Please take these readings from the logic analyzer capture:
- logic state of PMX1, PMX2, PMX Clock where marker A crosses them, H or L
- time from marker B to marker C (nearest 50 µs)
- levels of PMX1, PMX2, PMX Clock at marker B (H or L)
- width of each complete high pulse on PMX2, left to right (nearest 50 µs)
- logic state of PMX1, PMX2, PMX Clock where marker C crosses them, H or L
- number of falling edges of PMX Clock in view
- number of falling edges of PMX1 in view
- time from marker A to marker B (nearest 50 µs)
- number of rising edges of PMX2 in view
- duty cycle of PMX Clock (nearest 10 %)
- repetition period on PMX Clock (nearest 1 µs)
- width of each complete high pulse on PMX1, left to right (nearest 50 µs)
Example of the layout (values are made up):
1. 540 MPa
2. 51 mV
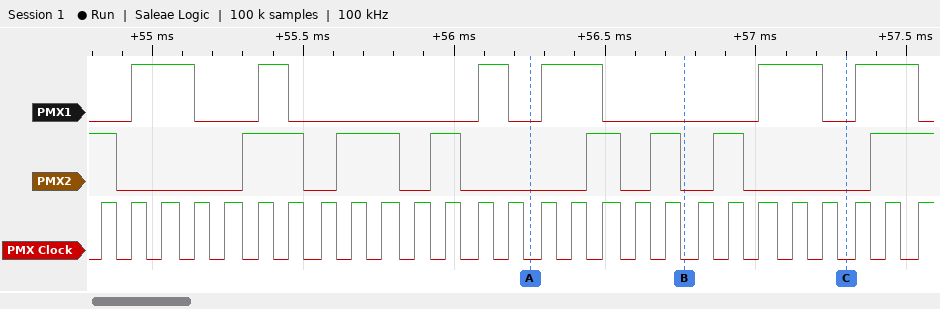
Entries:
1. PMX1=L, PMX2=L, PMX Clock=L
2. 550 µs
3. PMX1=L, PMX2=L, PMX Clock=L
4. 200 µs, 200 µs, 100 µs, 100 µs, 100 µs, 100 µs
5. PMX1=L, PMX2=L, PMX Clock=L
6. 26
7. 6
8. 500 µs
9. 7
10. 50 %
11. 104 µs
12. 200 µs, 100 µs, 100 µs, 200 µs, 200 µs, 200 µs
